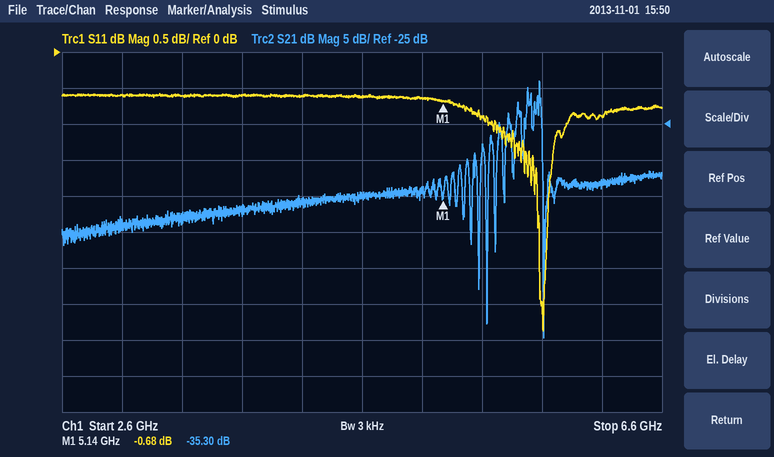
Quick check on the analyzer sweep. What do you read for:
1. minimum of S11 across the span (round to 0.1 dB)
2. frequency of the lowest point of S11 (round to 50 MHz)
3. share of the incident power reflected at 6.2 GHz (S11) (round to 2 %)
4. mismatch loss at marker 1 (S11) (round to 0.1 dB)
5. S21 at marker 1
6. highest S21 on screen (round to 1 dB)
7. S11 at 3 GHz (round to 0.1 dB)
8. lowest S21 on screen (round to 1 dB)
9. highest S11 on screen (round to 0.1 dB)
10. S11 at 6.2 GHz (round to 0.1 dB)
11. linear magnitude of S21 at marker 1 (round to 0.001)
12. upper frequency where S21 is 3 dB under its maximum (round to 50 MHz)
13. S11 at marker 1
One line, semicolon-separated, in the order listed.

-3.9 dB; 5.80 GHz; 82 %; 8.4 dB; -35.30 dB; -19 dB; -0.6 dB; -55 dB; -0.6 dB; -0.9 dB; 0.017; 5.80 GHz; -0.68 dB
